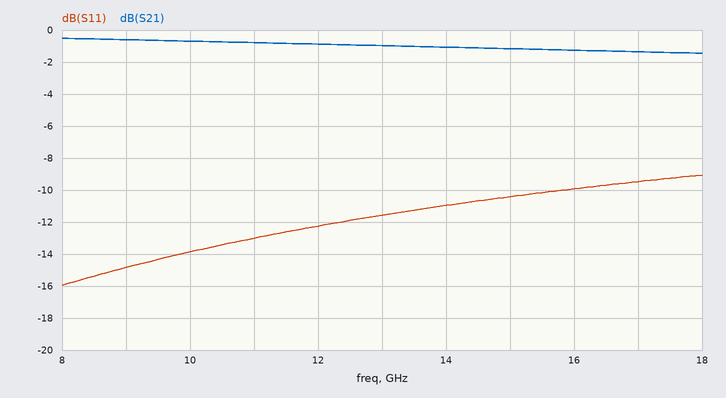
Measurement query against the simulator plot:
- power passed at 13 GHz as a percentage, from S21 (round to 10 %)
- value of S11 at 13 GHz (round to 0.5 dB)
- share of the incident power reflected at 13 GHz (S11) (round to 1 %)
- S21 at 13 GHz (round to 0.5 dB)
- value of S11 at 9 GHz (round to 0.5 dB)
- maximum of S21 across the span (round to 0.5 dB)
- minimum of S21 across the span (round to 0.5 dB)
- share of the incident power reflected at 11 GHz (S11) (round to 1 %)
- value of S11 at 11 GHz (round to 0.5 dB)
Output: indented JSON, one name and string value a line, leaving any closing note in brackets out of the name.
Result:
{
  "power passed at 13 GHz as a percentage, from S21": "80 %",
  "value of S11 at 13 GHz": "-11.5 dB",
  "share of the incident power reflected at 13 GHz (S11)": "7 %",
  "S21 at 13 GHz": "-1.0 dB",
  "value of S11 at 9 GHz": "-15.0 dB",
  "maximum of S21 across the span": "-0.5 dB",
  "minimum of S21 across the span": "-1.5 dB",
  "share of the incident power reflected at 11 GHz (S11)": "5 %",
  "value of S11 at 11 GHz": "-13.0 dB"
}
